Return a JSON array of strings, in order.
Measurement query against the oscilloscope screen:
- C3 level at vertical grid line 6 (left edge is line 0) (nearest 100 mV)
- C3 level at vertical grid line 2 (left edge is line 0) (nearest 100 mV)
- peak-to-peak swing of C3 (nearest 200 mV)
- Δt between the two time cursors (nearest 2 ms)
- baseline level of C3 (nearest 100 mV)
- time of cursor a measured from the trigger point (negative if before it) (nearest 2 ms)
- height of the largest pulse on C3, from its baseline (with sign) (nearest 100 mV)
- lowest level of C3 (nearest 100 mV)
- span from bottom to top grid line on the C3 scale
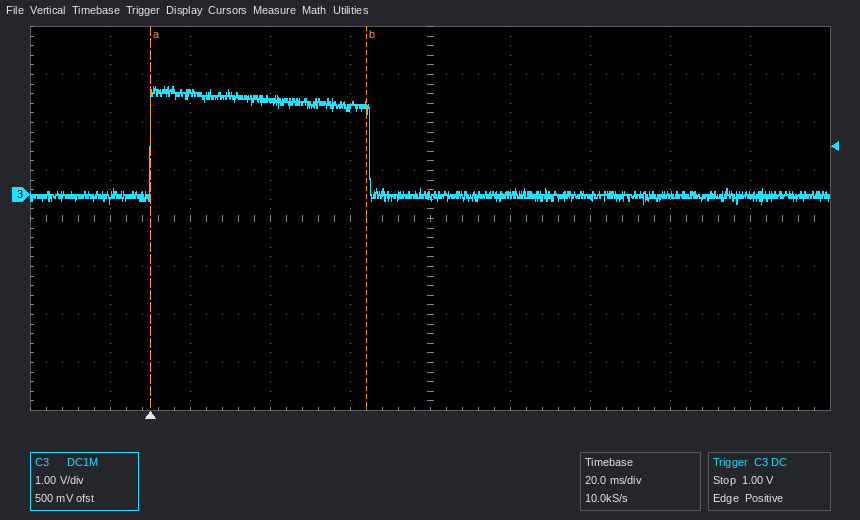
["0.0 V", "2.1 V", "2.4 V", "54 ms", "0.0 V", "0 ms", "+2.3 V", "-200 mV", "8 V"]
